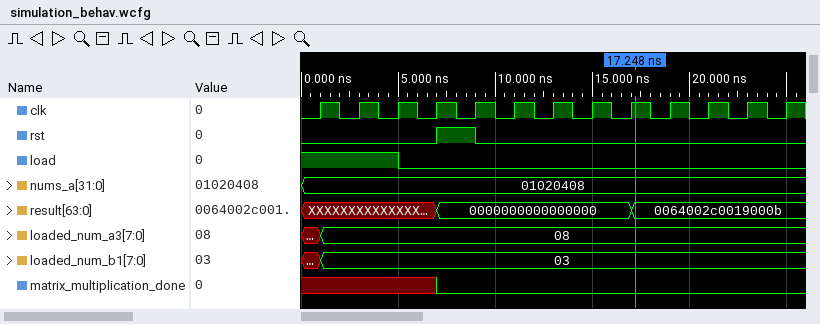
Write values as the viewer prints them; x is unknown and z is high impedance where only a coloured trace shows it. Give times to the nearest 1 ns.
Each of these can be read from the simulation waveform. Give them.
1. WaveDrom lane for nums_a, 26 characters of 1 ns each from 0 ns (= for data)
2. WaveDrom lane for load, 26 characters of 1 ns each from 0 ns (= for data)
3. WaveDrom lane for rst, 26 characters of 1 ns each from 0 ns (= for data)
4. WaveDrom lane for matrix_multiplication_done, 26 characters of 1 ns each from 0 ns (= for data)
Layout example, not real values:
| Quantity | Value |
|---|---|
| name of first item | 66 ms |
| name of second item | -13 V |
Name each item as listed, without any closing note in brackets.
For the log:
| Quantity | Value |
|---|---|
| WaveDrom lane for nums_a, 26 characters of 1 ns each from 0 ns | {name: 'nums_a', wave: '=.........................', data: '01020408'} |
| WaveDrom lane for load, 26 characters of 1 ns each from 0 ns | {name: 'load', wave: '1....0....................'} |
| WaveDrom lane for rst, 26 characters of 1 ns each from 0 ns | {name: 'rst', wave: '0......1.0................'} |
| WaveDrom lane for matrix_multiplication_done, 26 characters of 1 ns each from 0 ns | {name: 'matrix_multiplication_done', wave: 'x......0..................'} |
